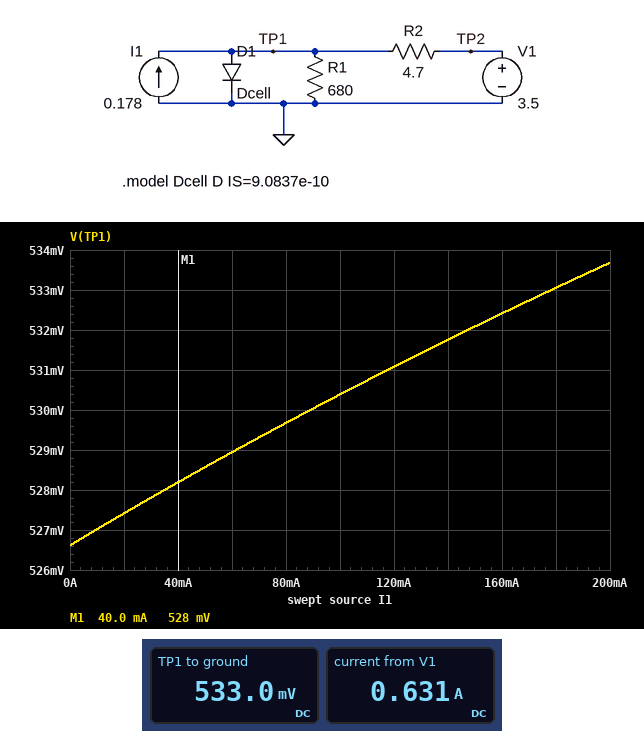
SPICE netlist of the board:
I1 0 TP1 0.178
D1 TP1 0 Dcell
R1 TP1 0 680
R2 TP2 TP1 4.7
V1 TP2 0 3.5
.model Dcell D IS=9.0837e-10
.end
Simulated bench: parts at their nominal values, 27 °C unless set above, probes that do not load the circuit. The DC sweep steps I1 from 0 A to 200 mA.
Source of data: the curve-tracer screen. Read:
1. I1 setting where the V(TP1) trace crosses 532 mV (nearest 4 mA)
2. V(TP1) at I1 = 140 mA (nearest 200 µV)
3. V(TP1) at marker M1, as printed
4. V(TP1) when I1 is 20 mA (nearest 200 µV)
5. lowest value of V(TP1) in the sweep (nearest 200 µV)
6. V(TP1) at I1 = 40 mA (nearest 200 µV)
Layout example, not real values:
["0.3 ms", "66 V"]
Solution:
["148 mA", "531.8 mV", "528 mV", "527.4 mV", "526.6 mV", "528.2 mV"]
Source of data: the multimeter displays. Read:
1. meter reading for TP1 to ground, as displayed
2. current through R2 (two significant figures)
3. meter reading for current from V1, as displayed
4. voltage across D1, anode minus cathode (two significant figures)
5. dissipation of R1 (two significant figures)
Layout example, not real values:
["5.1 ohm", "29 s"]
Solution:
["533.0 mV", "630 mA", "0.631 A", "530 mV", "420 µW"]
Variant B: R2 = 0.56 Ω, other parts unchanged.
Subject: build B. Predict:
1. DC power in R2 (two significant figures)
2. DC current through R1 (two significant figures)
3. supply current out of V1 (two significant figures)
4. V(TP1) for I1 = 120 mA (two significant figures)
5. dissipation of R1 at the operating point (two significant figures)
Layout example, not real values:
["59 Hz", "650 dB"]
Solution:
["15 W", "860 µA", "5.2 A", "580 mV", "500 µW"]
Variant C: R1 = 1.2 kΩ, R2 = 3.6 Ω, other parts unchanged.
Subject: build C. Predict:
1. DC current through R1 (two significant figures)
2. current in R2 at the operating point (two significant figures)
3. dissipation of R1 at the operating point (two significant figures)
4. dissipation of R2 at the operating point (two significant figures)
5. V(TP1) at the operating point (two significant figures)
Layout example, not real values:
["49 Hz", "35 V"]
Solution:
["450 µA", "820 mA", "240 µW", "2.4 W", "540 mV"]
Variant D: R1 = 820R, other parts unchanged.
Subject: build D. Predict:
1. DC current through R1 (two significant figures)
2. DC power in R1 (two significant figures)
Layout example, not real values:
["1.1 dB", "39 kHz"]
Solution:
["650 µA", "350 µW"]
